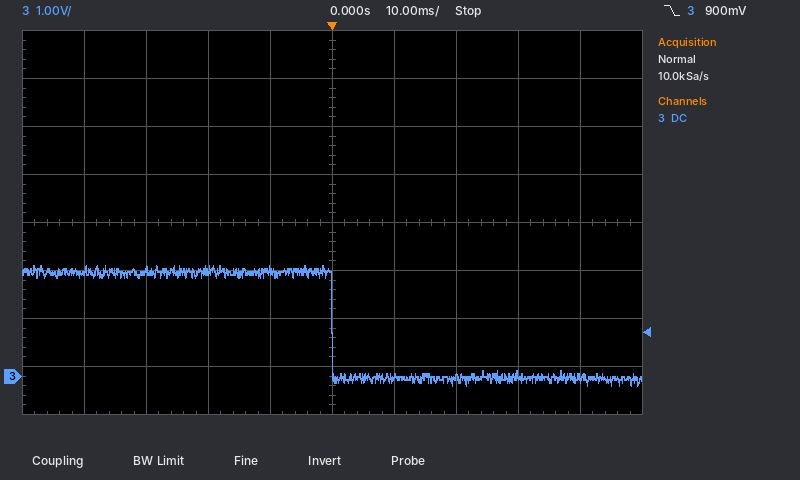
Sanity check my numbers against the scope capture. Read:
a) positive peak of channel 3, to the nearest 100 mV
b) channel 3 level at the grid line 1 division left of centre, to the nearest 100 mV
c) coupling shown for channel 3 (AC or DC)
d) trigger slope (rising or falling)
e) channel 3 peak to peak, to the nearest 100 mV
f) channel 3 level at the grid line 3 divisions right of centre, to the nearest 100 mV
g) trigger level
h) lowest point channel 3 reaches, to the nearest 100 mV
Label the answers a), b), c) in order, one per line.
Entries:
a) 2.3 V
b) 2.2 V
c) DC
d) falling
e) 2.5 V
f) 0.0 V
g) 900 mV
h) -200 mV
